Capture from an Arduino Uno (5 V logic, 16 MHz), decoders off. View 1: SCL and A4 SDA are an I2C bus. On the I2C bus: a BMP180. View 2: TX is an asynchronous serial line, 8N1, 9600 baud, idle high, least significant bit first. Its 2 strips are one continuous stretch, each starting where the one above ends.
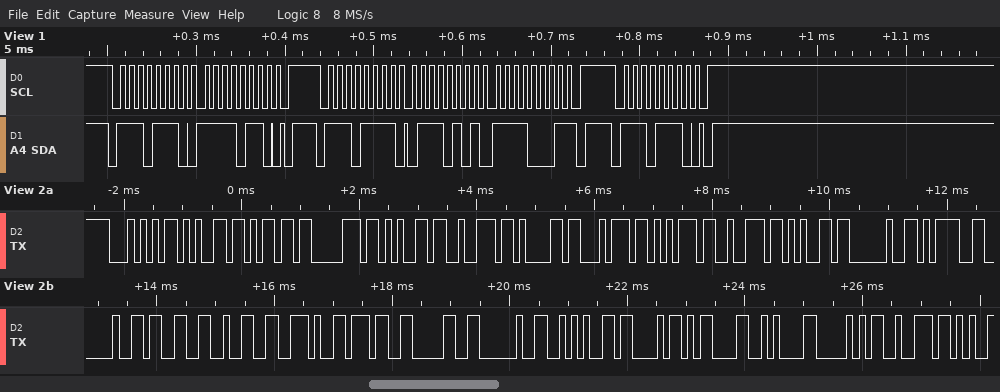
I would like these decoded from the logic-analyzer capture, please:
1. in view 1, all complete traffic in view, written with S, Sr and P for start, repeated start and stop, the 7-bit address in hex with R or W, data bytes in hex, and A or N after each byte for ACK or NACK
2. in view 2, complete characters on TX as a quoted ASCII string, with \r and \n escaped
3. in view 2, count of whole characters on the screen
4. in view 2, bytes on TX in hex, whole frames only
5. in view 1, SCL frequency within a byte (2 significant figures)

S 77W A F6 A P S 77R A 75 A F1 N P S 77W A P
"Temperature = 32.70 *C\r\nPr"
26
54 65 6D 70 65 72 61 74 75 72 65 20 3D 20 33 32 2E 37 30 20 2A 43 0D 0A 50 72
100 kHz
